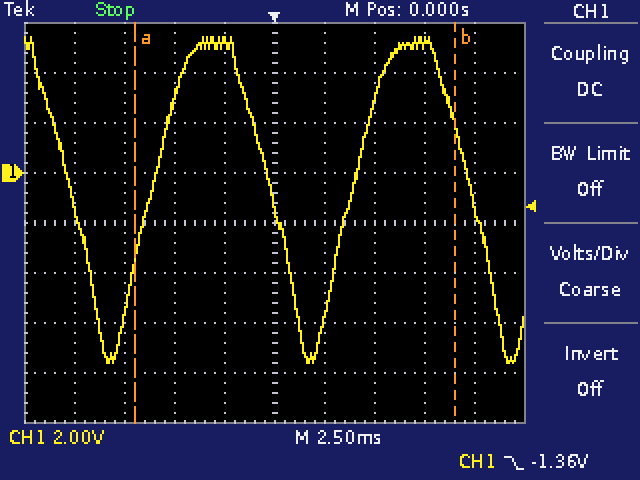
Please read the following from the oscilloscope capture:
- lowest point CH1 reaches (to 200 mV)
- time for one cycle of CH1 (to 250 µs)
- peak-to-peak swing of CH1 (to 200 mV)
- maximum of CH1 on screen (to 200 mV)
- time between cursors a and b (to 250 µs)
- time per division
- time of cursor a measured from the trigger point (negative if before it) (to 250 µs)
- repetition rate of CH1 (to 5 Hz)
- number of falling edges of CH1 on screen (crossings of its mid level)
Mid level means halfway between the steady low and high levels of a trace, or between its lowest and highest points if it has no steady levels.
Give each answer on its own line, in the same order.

-7.6 V
10.00 ms
13.0 V
5.4 V
16.00 ms
2.5 ms
-7.00 ms
100 Hz
3
